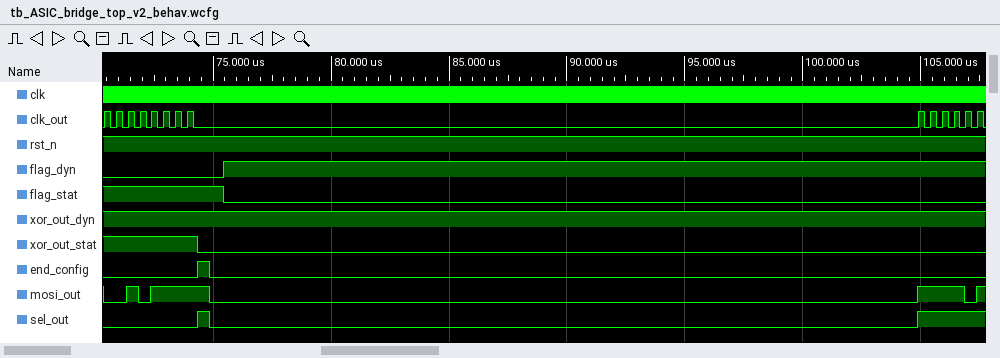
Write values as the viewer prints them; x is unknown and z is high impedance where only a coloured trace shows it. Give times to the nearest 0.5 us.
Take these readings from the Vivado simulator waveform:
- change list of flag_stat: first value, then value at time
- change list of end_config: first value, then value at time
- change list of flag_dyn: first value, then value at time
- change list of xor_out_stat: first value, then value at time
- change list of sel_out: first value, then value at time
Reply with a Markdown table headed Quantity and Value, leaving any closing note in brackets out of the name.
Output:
| Quantity | Value |
|---|---|
| change list of flag_stat: first value, then value at time | 1, 0 at 75.5 us |
| change list of end_config: first value, then value at time | 0, 1 at 74.5 us, 0 at 75 us |
| change list of flag_dyn: first value, then value at time | 0, 1 at 75.5 us |
| change list of xor_out_stat: first value, then value at time | 1, 0 at 74.5 us |
| change list of sel_out: first value, then value at time | 0, 1 at 74.5 us, 0 at 75 us, 1 at 105 us |
